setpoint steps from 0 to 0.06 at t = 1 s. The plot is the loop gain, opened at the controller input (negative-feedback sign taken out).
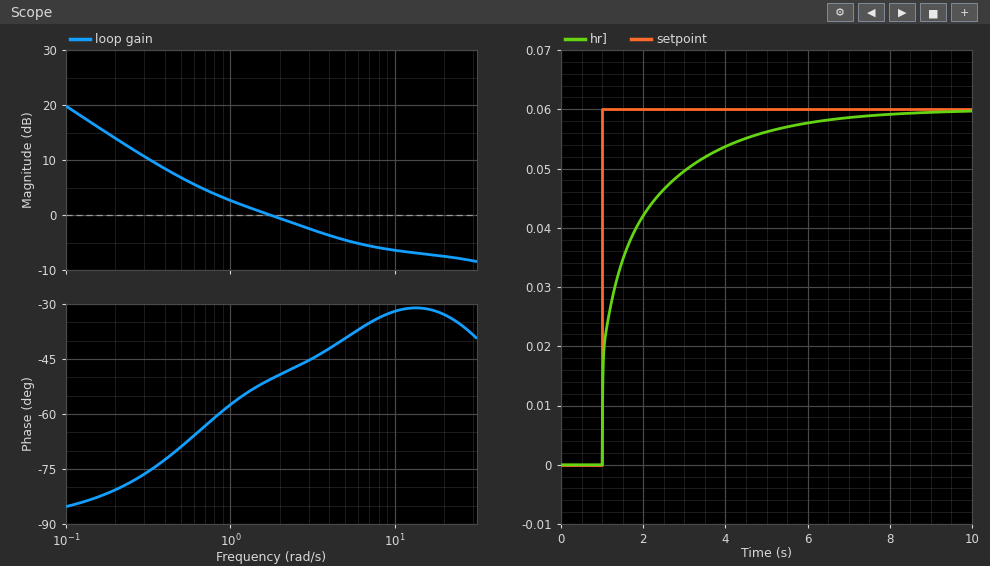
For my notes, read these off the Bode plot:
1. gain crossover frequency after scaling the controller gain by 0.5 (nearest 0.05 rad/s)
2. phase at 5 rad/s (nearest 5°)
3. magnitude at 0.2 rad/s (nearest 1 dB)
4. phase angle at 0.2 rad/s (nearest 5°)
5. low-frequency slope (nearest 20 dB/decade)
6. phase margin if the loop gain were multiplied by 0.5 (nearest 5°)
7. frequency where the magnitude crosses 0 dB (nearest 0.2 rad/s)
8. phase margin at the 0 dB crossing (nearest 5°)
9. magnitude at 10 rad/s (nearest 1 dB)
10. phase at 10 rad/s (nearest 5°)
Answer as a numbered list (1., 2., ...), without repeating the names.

1. 0.55 rad/s
2. -40°
3. 14 dB
4. -80°
5. -20 dB/decade
6. 115°
7. 1.8 rad/s
8. 130°
9. -6 dB
10. -30°
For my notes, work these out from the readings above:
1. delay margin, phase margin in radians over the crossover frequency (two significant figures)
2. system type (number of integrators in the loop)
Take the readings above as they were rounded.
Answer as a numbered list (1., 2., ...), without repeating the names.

1. 1.3 s
2. 1
